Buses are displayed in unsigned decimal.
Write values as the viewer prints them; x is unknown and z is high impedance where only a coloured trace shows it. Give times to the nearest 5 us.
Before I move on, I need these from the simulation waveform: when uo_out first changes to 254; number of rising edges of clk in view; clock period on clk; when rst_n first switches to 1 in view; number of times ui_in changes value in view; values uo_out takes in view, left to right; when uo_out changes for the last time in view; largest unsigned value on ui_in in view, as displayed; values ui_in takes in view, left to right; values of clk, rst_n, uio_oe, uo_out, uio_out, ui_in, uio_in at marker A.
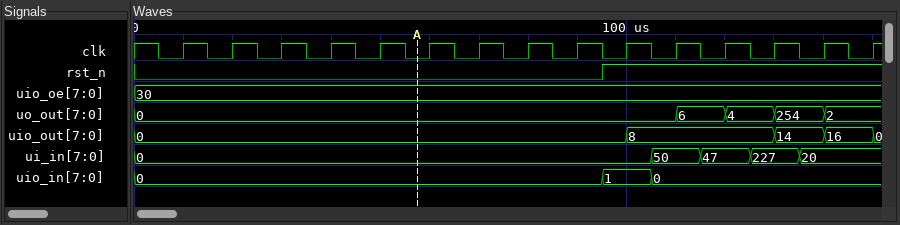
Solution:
130 us
15
10 us
95 us
4
0, 6, 4, 254, 2
140 us
227
0, 50, 47, 227, 20
clk=0, rst_n=0, uio_oe=30, uo_out=0, uio_out=0, ui_in=0, uio_in=0
